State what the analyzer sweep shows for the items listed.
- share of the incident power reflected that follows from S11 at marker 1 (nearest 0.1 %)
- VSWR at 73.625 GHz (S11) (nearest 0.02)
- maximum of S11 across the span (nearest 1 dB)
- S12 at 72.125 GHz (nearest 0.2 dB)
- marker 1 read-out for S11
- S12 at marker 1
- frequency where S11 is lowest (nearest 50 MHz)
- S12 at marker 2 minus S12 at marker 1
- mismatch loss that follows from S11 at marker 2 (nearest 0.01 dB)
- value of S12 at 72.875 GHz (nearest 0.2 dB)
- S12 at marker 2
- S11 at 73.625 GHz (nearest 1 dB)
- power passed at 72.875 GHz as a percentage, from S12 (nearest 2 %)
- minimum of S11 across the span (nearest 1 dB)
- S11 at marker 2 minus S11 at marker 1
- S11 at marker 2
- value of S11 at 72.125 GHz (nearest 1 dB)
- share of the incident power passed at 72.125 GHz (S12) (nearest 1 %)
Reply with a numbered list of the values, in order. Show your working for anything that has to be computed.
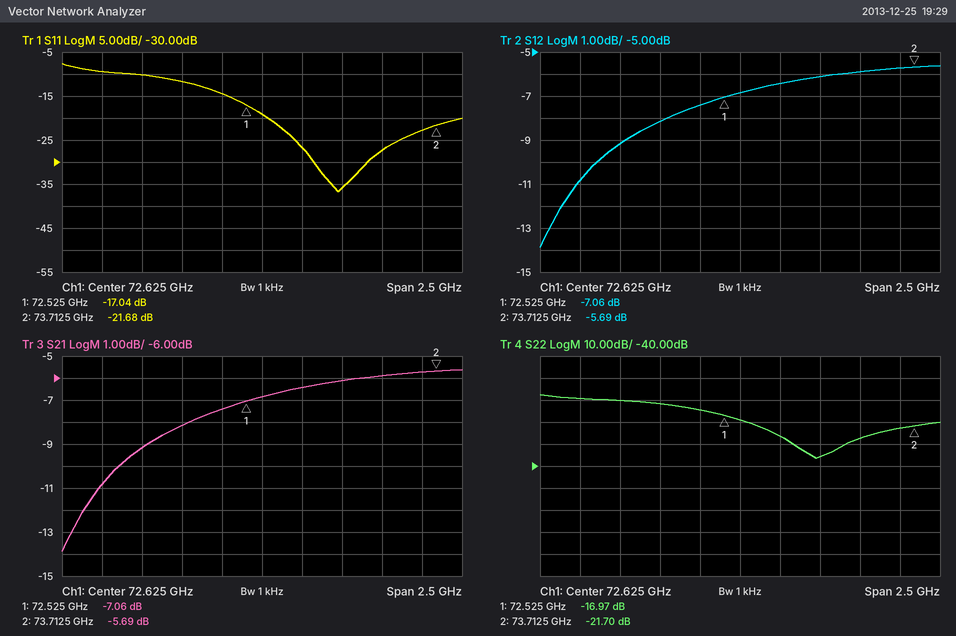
1. 10^(-17.04/10) ≈ 2.0 %
2. |Γ| = 10^(-23/20) = 0.0708; VSWR = (1 + 0.0708)/(1 − 0.0708) ≈ 1.15, so 1.16 to the nearest 0.02
3. -8 dB
4. -8.2 dB
5. -17.04 dB
6. -7.06 dB
7. 73.10 GHz
8. -5.69 − (-7.06) = 1.37 dB
9. −10 log10(1 − 10^(-21.68/10)) ≈ 0.03 dB
10. -6.4 dB
11. -5.69 dB
12. -23 dB
13. 10^(-6.4/10) ≈ 22.9 %, so 22 % to the nearest 2 %
14. -37 dB
15. -21.68 − (-17.04) = -4.64 dB
16. -21.68 dB
17. -12 dB
18. 10^(-8.2/10) ≈ 15 %
